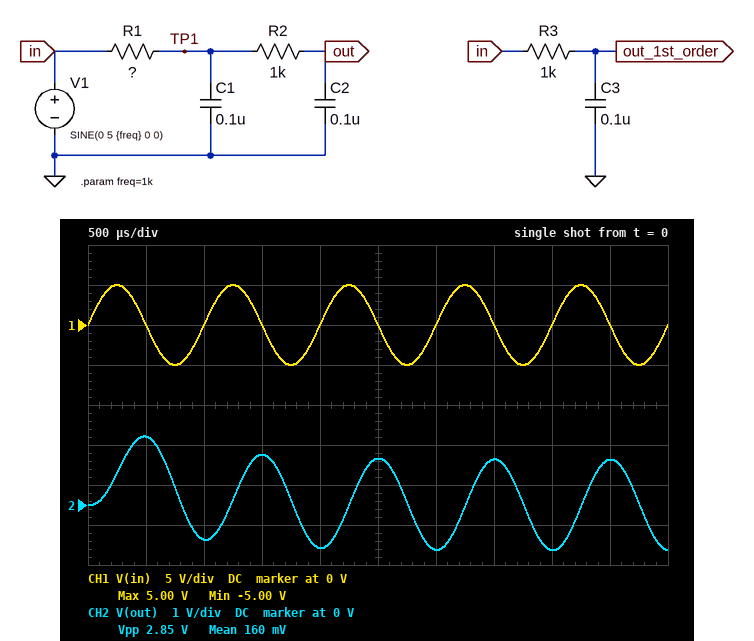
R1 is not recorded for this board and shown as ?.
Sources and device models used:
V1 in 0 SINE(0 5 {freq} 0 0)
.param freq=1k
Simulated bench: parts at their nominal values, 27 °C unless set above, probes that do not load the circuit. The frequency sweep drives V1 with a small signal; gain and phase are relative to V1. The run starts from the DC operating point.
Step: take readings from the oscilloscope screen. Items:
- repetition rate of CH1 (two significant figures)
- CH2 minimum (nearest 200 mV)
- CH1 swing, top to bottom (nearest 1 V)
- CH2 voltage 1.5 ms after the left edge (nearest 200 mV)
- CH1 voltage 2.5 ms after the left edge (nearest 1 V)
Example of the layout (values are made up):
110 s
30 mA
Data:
1.0 kHz
-1.2 V
10 V
1.2 V
0 V
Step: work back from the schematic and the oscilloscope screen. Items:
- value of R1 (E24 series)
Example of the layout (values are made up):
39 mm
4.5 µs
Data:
3 kΩ
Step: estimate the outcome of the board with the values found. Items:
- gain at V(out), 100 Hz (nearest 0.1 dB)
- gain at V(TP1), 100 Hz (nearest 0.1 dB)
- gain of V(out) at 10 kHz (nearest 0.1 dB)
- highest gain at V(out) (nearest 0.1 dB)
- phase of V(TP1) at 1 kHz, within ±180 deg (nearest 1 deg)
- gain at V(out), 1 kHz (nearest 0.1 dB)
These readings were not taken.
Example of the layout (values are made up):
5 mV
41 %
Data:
-0.7 dB
-0.7 dB
-42.0 dB
0 dB
-60 deg
-12.9 dB
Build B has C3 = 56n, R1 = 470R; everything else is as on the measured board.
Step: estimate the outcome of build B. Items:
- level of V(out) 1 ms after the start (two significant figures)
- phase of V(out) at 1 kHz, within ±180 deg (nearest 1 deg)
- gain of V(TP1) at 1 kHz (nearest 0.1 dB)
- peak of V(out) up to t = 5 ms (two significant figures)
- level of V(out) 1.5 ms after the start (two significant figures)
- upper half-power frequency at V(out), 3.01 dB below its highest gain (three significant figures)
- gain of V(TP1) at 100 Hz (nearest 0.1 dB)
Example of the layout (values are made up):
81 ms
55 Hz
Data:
-2.8 V
-56 deg
-1.9 dB
3.7 V
2.8 V
935 Hz
0 dB
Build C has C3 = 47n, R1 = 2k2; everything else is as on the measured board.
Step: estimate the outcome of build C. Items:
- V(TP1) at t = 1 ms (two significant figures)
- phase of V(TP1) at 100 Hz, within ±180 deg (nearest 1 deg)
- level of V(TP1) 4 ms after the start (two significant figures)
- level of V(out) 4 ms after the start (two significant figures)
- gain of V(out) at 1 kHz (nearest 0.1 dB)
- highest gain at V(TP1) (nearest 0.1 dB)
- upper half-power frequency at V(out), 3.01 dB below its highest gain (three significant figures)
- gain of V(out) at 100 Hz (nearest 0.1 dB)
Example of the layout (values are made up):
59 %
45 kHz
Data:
-1.3 V
-15 deg
-1.4 V
-1.5 V
-10.6 dB
0 dB
319 Hz
-0.4 dB
